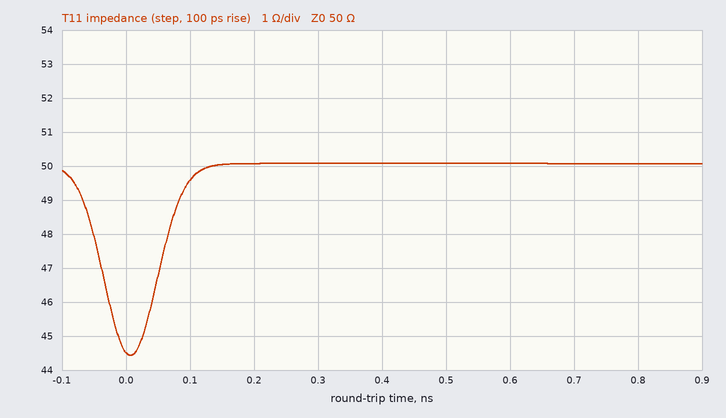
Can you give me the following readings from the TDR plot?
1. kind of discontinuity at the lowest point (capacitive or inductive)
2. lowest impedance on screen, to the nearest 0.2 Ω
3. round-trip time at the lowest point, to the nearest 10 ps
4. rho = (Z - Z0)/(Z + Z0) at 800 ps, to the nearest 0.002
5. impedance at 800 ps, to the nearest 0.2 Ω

capacitive
44.4 Ω
10 ps
0.000
50.0 Ω
